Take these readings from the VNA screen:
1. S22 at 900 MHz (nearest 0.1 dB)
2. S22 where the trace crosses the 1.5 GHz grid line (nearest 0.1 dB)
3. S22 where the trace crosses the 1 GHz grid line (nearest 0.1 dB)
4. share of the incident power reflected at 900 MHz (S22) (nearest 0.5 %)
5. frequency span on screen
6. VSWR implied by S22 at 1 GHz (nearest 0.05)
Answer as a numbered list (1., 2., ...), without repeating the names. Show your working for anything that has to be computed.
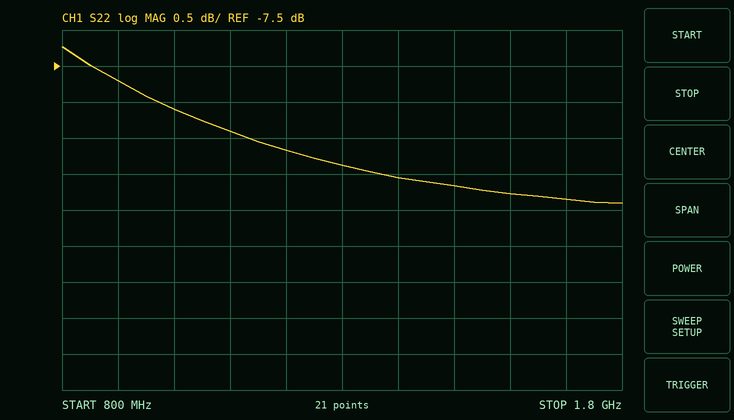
1. -7.7 dB
2. -9.2 dB
3. -8.1 dB
4. 10^(-7.7/10) ≈ 17.0 %
5. 1 GHz
6. |Γ| = 10^(-8.1/20) = 0.3936; VSWR = (1 + 0.3936)/(1 − 0.3936) ≈ 2.30
